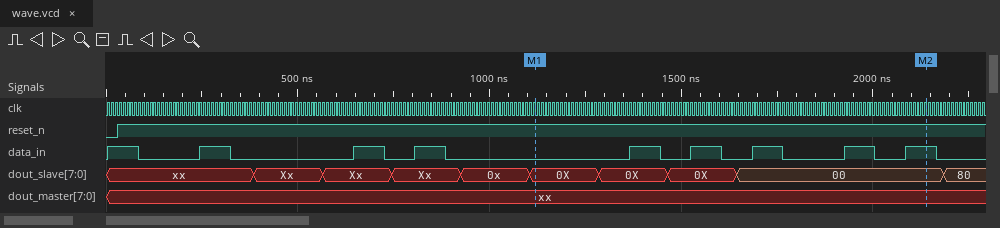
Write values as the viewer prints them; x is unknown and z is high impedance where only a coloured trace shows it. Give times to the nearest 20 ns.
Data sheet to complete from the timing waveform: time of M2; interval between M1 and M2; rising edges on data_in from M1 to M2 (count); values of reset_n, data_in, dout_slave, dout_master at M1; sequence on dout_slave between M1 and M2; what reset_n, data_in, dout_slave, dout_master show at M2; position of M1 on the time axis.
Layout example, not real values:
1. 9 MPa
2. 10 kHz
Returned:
1. 2140 ns
2. 1020 ns
3. 5
4. reset_n=1, data_in=0, dout_slave=0X, dout_master=xx
5. 0X, 0X, 0X, 00
6. reset_n=1, data_in=1, dout_slave=00, dout_master=xx
7. 1120 ns
